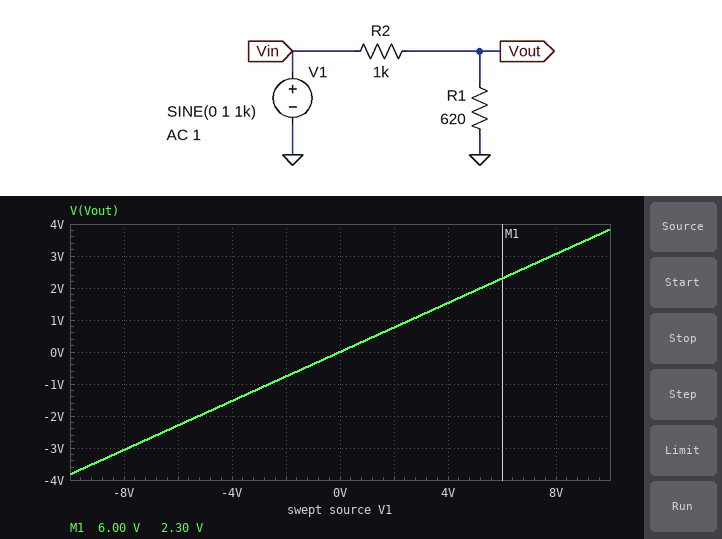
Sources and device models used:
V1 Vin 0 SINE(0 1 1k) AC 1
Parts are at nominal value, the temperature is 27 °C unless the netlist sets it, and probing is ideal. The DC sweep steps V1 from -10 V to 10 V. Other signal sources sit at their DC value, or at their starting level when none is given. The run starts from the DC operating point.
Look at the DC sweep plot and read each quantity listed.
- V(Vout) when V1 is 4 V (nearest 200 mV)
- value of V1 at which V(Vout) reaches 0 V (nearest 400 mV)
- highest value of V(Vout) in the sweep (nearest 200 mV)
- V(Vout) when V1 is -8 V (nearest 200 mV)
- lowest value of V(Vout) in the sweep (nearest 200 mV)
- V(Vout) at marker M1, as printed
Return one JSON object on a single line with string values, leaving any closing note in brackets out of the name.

{"V(Vout) when V1 is 4 V": "1.6 V", "value of V1 at which V(Vout) reaches 0 V": "0 V", "highest value of V(Vout) in the sweep": "3.8 V", "V(Vout) when V1 is -8 V": "-3.0 V", "lowest value of V(Vout) in the sweep": "-3.8 V", "V(Vout) at marker M1, as printed": "2.30 V"}
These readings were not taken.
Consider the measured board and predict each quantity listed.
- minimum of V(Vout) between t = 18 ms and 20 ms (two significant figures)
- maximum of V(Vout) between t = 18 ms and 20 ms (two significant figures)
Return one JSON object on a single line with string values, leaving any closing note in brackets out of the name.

{"minimum of V(Vout) between t = 18 ms and 20 ms": "-380 mV", "maximum of V(Vout) between t = 18 ms and 20 ms": "380 mV"}
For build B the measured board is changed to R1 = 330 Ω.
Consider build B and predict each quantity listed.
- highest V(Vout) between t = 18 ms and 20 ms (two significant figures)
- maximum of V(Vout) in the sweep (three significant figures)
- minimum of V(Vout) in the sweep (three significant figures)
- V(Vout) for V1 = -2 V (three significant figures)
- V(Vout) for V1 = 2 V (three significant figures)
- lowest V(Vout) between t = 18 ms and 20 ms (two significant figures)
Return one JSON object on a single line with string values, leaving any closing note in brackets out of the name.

{"highest V(Vout) between t = 18 ms and 20 ms": "250 mV", "maximum of V(Vout) in the sweep": "2.48 V", "minimum of V(Vout) in the sweep": "-2.48 V", "V(Vout) for V1 = -2 V": "-496 mV", "V(Vout) for V1 = 2 V": "496 mV", "lowest V(Vout) between t = 18 ms and 20 ms": "-250 mV"}
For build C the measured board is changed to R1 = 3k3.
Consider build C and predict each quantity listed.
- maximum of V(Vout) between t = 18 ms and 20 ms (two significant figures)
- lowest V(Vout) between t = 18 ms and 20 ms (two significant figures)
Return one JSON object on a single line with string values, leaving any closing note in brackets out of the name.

{"maximum of V(Vout) between t = 18 ms and 20 ms": "770 mV", "lowest V(Vout) between t = 18 ms and 20 ms": "-770 mV"}
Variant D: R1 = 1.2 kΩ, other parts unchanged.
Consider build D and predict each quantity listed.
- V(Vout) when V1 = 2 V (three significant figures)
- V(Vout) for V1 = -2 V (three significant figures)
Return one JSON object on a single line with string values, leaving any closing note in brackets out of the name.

{"V(Vout) when V1 = 2 V": "1.09 V", "V(Vout) for V1 = -2 V": "-1.09 V"}
